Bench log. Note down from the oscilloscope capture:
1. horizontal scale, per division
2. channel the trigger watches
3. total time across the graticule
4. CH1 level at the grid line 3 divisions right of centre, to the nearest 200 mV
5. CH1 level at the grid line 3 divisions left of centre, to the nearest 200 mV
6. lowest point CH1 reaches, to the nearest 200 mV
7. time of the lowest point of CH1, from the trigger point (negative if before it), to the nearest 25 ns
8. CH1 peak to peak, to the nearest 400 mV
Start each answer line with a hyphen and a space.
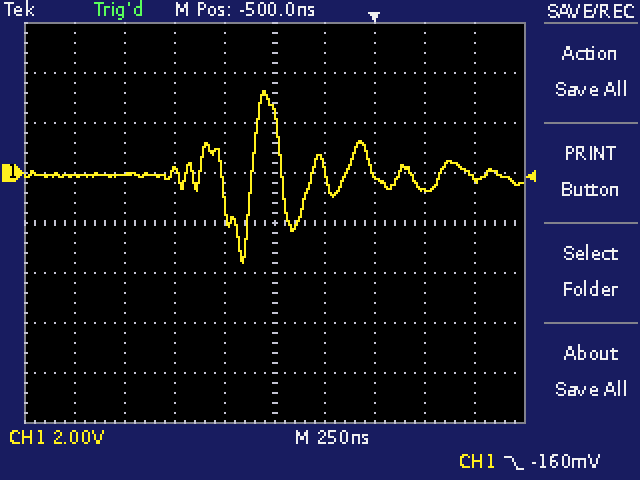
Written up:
- 250 ns
- CH1
- 2.5 µs
- -600 mV
- 0.0 V
- -3.6 V
- -650 ns
- 6.8 V
